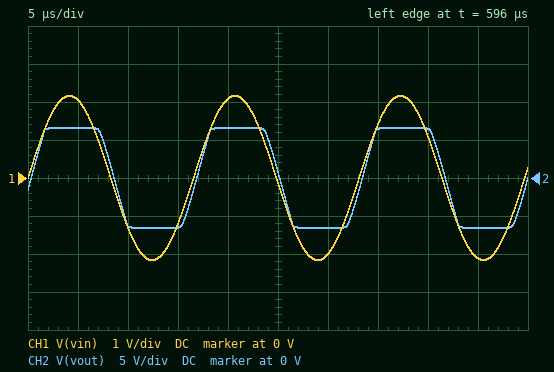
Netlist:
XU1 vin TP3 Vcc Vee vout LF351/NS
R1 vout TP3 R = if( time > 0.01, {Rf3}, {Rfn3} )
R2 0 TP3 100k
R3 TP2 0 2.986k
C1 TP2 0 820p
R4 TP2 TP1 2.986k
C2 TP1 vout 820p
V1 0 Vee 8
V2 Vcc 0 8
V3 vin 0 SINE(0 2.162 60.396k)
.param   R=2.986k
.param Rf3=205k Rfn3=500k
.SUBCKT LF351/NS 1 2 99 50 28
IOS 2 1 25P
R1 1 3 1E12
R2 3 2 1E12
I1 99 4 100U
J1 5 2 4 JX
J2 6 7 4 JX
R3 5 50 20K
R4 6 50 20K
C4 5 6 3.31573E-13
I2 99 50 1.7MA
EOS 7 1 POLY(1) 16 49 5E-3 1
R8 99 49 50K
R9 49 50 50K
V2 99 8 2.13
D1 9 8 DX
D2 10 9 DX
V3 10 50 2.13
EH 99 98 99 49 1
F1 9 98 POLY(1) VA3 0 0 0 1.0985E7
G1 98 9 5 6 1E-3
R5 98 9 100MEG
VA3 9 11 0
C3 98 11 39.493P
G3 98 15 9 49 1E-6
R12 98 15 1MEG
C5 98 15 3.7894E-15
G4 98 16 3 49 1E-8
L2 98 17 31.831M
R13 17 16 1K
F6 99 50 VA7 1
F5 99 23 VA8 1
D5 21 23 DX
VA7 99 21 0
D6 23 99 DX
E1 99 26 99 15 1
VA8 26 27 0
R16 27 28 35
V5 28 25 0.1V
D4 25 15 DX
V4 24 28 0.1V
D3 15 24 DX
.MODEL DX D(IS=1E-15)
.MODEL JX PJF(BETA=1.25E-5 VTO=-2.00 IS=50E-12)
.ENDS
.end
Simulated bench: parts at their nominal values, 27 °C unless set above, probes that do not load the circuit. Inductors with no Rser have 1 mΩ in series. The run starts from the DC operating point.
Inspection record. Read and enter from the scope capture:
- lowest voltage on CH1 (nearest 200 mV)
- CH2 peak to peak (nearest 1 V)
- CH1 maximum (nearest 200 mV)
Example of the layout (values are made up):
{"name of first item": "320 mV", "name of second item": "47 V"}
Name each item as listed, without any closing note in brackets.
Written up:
{"lowest voltage on CH1": "-2.2 V", "CH2 peak to peak": "13 V", "CH1 maximum": "2.2 V"}
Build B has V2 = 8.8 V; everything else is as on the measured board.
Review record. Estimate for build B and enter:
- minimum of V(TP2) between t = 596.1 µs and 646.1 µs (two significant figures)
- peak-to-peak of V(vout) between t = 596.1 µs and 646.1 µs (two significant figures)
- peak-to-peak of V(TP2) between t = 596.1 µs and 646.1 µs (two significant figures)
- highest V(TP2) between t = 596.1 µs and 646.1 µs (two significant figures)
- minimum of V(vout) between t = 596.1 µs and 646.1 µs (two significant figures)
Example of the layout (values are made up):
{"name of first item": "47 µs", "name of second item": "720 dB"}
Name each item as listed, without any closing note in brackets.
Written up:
{"minimum of V(TP2) between t = 596.1 µs and 646.1 µs": "-2.7 V", "peak-to-peak of V(vout) between t = 596.1 µs and 646.1 µs": "14 V", "peak-to-peak of V(TP2) between t = 596.1 µs and 646.1 µs": "5.4 V", "highest V(TP2) between t = 596.1 µs and 646.1 µs": "2.7 V", "minimum of V(vout) between t = 596.1 µs and 646.1 µs": "-6.6 V"}
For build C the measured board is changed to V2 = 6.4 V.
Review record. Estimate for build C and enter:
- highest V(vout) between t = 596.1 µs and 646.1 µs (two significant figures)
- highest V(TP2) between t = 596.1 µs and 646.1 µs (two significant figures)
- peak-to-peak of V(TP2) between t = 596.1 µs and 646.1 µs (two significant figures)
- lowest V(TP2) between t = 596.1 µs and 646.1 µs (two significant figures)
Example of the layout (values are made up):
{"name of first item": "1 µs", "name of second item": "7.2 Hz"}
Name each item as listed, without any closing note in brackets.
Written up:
{"highest V(vout) between t = 596.1 µs and 646.1 µs": "5.0 V", "highest V(TP2) between t = 596.1 µs and 646.1 µs": "2.2 V", "peak-to-peak of V(TP2) between t = 596.1 µs and 646.1 µs": "4.6 V", "lowest V(TP2) between t = 596.1 µs and 646.1 µs": "-2.3 V"}
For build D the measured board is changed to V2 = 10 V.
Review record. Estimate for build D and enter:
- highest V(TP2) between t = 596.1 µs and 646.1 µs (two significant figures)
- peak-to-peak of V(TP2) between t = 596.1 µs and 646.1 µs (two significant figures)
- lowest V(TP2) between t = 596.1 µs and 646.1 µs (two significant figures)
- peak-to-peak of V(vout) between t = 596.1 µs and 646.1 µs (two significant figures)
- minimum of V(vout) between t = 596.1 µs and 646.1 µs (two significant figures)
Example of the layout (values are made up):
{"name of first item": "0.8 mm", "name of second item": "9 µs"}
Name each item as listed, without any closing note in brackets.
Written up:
{"highest V(TP2) between t = 596.1 µs and 646.1 µs": "3.0 V", "peak-to-peak of V(TP2) between t = 596.1 µs and 646.1 µs": "5.8 V", "lowest V(TP2) between t = 596.1 µs and 646.1 µs": "-2.8 V", "peak-to-peak of V(vout) between t = 596.1 µs and 646.1 µs": "15 V", "minimum of V(vout) between t = 596.1 µs and 646.1 µs": "-6.6 V"}
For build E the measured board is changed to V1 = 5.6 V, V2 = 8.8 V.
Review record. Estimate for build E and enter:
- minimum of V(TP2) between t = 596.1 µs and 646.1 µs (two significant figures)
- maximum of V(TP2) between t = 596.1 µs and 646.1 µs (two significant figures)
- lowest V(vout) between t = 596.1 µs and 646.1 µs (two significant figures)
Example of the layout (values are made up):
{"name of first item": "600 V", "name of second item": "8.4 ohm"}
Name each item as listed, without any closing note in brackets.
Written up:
{"minimum of V(TP2) between t = 596.1 µs and 646.1 µs": "-2.2 V", "maximum of V(TP2) between t = 596.1 µs and 646.1 µs": "2.4 V", "lowest V(vout) between t = 596.1 µs and 646.1 µs": "-4.2 V"}
